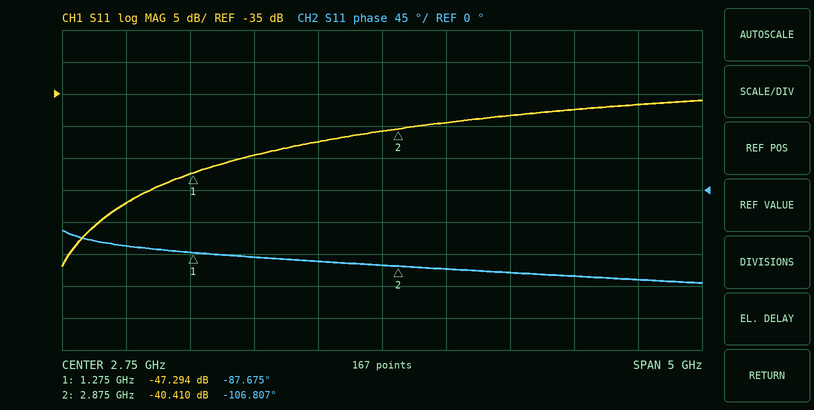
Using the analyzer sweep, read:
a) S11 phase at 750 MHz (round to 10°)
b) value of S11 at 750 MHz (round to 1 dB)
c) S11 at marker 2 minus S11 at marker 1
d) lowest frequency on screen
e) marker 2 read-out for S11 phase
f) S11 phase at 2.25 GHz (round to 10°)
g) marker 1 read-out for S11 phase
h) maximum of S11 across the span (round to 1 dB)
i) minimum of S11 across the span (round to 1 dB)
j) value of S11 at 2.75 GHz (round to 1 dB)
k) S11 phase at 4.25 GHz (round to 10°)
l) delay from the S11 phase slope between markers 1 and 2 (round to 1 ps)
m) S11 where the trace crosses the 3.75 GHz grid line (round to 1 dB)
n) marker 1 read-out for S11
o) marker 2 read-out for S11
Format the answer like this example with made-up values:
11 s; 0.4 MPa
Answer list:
-80°; -52 dB; 6.884 dB; 250 MHz; -106.807°; -100°; -87.675°; -36 dB; -62 dB; -41 dB; -120°; 33 ps; -38 dB; -47.294 dB; -40.410 dB
